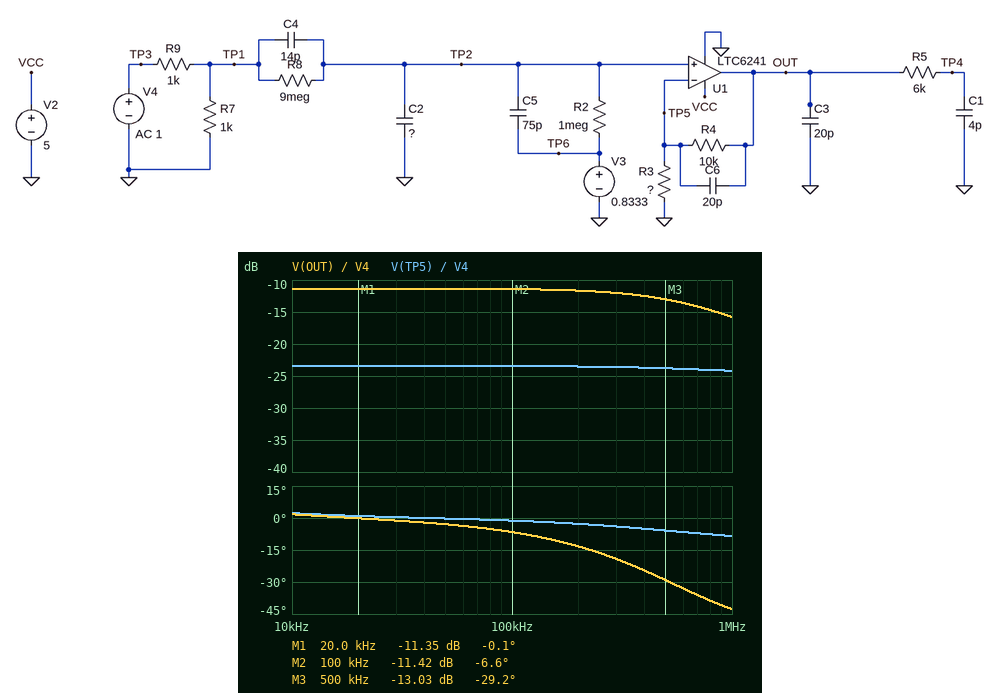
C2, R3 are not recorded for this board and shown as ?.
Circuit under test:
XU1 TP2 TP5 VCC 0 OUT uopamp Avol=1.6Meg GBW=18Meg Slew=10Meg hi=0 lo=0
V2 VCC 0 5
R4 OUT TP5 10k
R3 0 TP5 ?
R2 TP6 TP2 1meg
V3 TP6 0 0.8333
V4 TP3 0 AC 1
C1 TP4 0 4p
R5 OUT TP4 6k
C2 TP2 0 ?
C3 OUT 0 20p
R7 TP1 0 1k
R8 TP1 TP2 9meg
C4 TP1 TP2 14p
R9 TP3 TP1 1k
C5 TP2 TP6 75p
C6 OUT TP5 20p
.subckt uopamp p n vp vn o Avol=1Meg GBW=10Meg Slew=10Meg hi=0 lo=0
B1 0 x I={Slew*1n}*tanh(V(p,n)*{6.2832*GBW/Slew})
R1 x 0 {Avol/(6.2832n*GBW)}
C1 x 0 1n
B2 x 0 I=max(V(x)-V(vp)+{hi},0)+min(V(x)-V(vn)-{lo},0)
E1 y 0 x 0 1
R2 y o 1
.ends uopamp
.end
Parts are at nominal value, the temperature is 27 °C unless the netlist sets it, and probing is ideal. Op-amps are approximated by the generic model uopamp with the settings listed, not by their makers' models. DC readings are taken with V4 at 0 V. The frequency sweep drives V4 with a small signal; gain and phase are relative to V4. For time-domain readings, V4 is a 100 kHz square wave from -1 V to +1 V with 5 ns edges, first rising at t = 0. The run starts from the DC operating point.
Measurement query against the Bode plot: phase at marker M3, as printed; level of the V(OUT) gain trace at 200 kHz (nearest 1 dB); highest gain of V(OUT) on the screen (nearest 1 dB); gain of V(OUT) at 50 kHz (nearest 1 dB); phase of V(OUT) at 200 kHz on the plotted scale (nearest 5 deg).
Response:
-29.2 deg
-12 dB
-11 dB
-11 dB
-15 deg
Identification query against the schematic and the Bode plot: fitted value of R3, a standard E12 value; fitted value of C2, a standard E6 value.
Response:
3.3 kΩ
15 pF
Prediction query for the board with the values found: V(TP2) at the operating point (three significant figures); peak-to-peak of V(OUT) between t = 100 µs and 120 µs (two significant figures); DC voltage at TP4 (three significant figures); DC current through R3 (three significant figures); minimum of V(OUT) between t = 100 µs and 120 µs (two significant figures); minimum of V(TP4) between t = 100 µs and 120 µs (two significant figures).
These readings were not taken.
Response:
750 mV
550 mV
3.02 V
227 µA
2.8 V
2.8 V
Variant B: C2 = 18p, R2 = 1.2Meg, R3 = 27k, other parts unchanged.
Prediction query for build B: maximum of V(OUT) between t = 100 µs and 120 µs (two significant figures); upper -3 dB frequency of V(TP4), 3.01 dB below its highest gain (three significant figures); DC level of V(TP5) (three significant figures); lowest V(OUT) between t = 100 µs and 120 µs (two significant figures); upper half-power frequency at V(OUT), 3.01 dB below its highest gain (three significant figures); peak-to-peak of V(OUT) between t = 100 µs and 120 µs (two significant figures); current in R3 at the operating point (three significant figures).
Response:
1.1 V
2.23 MHz
735 mV
920 mV
3.90 MHz
180 mV
27.2 µA
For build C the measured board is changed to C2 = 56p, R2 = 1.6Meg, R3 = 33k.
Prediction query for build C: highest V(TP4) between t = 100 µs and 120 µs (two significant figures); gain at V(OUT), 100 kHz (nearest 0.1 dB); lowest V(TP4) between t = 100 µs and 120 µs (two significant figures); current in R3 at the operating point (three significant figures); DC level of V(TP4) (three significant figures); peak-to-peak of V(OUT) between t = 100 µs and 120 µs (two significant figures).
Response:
970 mV
-24.1 dB
840 mV
21.4 µA
922 mV
130 mV
